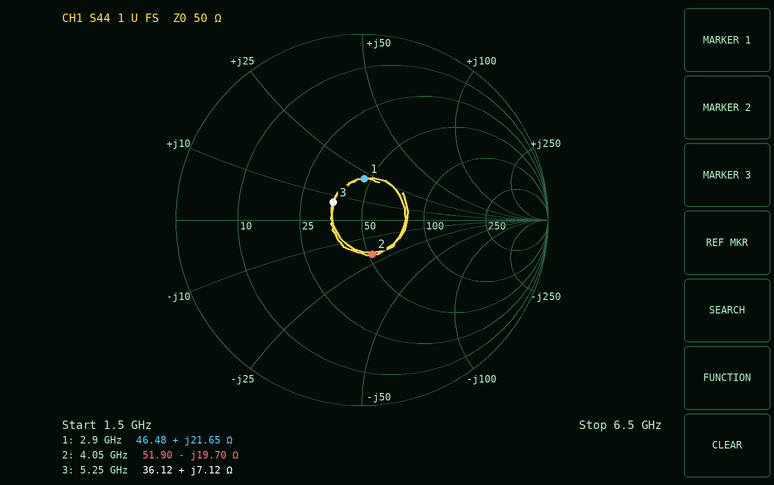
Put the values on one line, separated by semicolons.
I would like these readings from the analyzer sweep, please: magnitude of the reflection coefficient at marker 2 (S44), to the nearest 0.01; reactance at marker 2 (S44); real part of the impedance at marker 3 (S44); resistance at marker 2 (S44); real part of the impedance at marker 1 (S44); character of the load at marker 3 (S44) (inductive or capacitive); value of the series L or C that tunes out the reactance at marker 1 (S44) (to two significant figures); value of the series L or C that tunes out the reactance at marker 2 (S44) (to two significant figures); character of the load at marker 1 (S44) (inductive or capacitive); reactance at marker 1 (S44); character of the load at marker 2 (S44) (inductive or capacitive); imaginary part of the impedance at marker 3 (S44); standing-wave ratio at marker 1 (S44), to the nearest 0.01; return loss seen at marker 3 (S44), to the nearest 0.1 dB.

0.19; -19.70 Ω; 36.12 Ω; 51.90 Ω; 46.48 Ω; inductive; 2.5 pF; 770 pH; inductive; +21.65 Ω; capacitive; +7.12 Ω; 1.57; 14.9 dB
